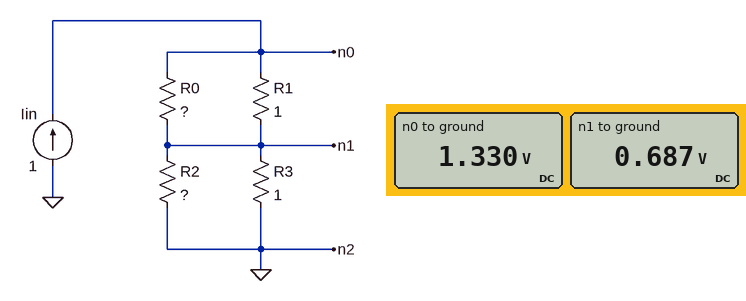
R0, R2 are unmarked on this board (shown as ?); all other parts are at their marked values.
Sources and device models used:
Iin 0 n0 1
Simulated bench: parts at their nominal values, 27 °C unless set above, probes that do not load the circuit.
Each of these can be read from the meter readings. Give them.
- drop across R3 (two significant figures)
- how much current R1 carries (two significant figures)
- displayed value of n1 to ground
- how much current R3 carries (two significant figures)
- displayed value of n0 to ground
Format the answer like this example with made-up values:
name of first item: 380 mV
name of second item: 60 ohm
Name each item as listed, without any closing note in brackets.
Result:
drop across R3: 690 mV
how much current R1 carries: 640 mA
displayed value of n1 to ground: 0.687 V
how much current R3 carries: 690 mA
displayed value of n0 to ground: 1.330 V
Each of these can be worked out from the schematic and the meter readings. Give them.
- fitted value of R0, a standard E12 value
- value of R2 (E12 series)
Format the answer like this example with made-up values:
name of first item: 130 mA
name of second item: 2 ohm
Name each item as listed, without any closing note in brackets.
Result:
fitted value of R0, a standard E12 value: 1.8 Ω
value of R2: 2.2 Ω
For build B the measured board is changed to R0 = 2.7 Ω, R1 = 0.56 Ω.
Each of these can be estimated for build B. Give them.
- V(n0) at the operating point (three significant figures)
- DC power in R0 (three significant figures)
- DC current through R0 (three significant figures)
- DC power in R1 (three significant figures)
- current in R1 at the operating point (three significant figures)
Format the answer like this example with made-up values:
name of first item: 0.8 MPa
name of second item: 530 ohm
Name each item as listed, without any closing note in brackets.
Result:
V(n0) at the operating point: 1.15 V
DC power in R0: 79.7 mW
DC current through R0: 172 mA
DC power in R1: 384 mW
current in R1 at the operating point: 828 mA
